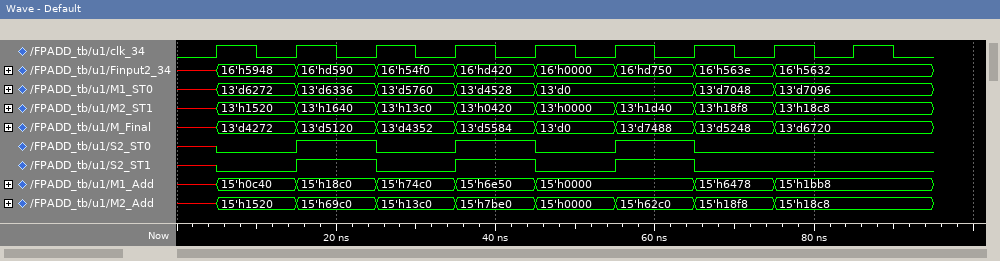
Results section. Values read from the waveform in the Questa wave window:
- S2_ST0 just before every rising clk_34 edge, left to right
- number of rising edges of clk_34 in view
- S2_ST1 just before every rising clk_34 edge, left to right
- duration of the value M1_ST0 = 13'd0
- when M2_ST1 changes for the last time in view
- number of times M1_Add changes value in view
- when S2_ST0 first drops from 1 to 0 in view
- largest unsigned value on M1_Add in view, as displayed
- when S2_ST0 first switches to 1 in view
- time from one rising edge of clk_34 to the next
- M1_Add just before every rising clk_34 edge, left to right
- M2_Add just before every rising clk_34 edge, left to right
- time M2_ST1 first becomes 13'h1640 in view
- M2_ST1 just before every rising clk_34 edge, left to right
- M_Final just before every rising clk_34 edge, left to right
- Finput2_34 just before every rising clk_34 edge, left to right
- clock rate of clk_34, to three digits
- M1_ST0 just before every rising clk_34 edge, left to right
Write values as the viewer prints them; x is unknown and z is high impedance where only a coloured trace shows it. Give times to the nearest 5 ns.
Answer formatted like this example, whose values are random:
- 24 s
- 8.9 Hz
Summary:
- x 0 1 0 1 0 1 0 0
- 9
- x 0 1 0 1 0 1 0 0
- 20 ns
- 75 ns
- 7
- 25 ns
- 15'h74c0
- 15 ns
- 10 ns
- x, 15'h0c40, 15'h18c0, 15'h74c0, 15'h6e50, 15'h0000, 15'h0000, 15'h6478, 15'h1bb8
- x, 15'h1520, 15'h69c0, 15'h13c0, 15'h7be0, 15'h0000, 15'h62c0, 15'h18f8, 15'h18c8
- 15 ns
- x, 13'h1520, 13'h1640, 13'h13c0, 13'h0420, 13'h0000, 13'h1d40, 13'h18f8, 13'h18c8
- x, 13'd4272, 13'd5120, 13'd4352, 13'd5584, 13'd0, 13'd7488, 13'd5248, 13'd6720
- x, 16'h5948, 16'hd590, 16'h54f0, 16'hd420, 16'h0000, 16'hd750, 16'h563e, 16'h5632
- 100 MHz
- x, 13'd6272, 13'd6336, 13'd5760, 13'd4528, 13'd0, 13'd0, 13'd7048, 13'd7096
